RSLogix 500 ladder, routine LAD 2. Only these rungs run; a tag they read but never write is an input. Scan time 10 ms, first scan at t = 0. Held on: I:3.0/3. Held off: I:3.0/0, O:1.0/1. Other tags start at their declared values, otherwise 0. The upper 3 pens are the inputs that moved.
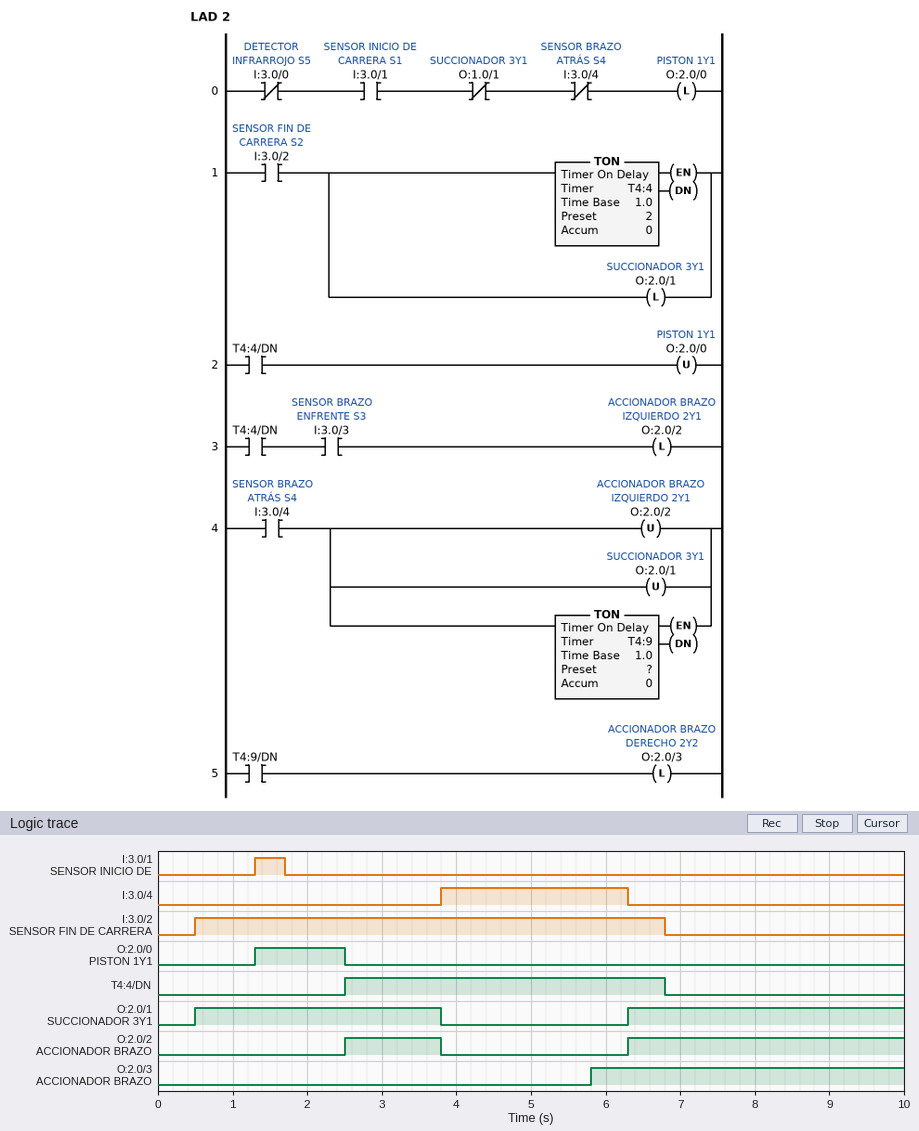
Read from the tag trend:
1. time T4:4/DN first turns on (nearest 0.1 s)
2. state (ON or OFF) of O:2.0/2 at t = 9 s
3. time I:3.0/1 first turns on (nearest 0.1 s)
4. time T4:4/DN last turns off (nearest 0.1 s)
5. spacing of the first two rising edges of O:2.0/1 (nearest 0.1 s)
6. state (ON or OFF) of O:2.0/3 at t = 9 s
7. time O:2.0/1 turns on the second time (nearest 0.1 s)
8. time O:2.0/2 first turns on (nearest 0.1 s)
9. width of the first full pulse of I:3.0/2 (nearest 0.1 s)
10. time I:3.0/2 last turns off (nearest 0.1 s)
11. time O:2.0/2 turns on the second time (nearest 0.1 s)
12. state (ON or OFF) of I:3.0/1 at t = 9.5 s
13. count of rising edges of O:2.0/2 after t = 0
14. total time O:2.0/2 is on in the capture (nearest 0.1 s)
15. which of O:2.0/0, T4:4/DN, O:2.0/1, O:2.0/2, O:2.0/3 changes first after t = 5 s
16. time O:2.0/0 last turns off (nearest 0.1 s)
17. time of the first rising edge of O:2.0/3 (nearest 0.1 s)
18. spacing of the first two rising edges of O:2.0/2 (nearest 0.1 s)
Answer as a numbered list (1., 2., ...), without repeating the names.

1. 2.5 s
2. ON
3. 1.3 s
4. 6.8 s
5. 5.8 s
6. ON
7. 6.3 s
8. 2.5 s
9. 6.3 s
10. 6.8 s
11. 6.3 s
12. OFF
13. 2
14. 5.0 s
15. O:2.0/3
16. 2.5 s
17. 5.8 s
18. 3.8 s
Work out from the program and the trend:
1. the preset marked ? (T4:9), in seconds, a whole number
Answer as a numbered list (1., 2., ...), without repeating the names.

1. 2 s
